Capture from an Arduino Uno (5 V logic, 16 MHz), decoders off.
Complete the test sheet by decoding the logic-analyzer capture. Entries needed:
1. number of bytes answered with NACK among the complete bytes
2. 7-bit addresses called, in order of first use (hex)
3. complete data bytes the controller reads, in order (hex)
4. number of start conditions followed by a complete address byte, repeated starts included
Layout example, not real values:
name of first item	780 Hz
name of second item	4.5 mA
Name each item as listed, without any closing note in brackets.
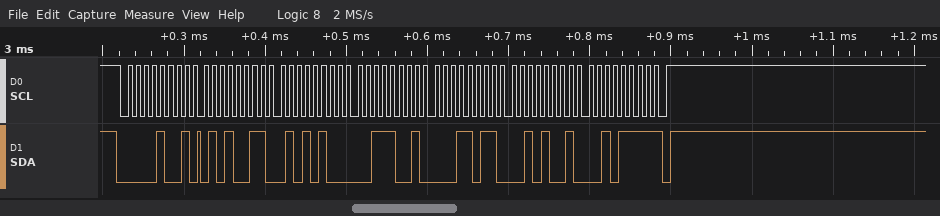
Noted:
number of bytes answered with NACK among the complete bytes	1
7-bit addresses called, in order of first use	0x04
complete data bytes the controller reads, in order	53 54 39 1B 29 2F
number of start conditions followed by a complete address byte, repeated starts included	1
